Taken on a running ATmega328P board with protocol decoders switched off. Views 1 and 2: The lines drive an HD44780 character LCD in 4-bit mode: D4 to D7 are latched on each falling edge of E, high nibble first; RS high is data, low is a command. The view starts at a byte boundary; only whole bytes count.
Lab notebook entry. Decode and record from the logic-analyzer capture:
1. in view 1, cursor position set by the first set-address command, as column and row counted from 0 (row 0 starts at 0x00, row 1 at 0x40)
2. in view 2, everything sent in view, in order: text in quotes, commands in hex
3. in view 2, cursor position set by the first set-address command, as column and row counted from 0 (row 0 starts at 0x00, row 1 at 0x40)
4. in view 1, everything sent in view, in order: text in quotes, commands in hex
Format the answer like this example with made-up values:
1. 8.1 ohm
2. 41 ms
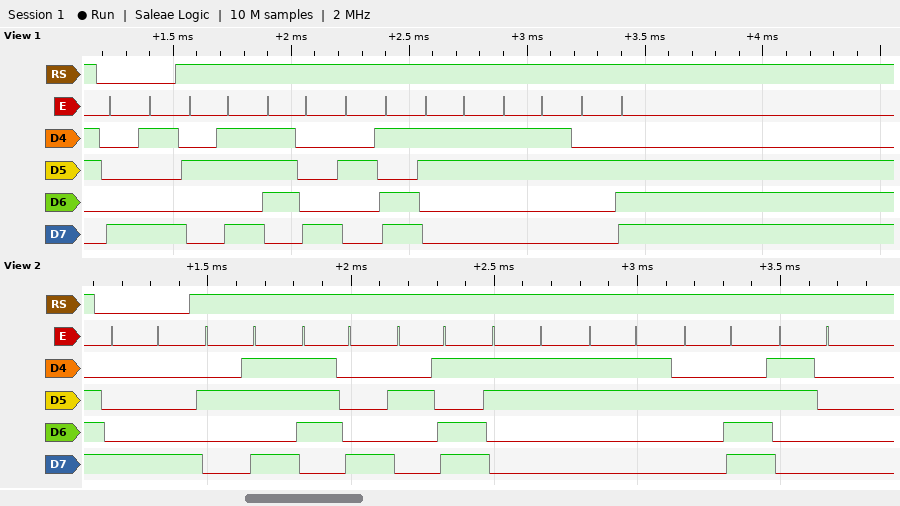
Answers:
1. column 9, row 0
2. 0x88 "+x-33.0"
3. column 8, row 0
4. 0x89 "+x-33."
